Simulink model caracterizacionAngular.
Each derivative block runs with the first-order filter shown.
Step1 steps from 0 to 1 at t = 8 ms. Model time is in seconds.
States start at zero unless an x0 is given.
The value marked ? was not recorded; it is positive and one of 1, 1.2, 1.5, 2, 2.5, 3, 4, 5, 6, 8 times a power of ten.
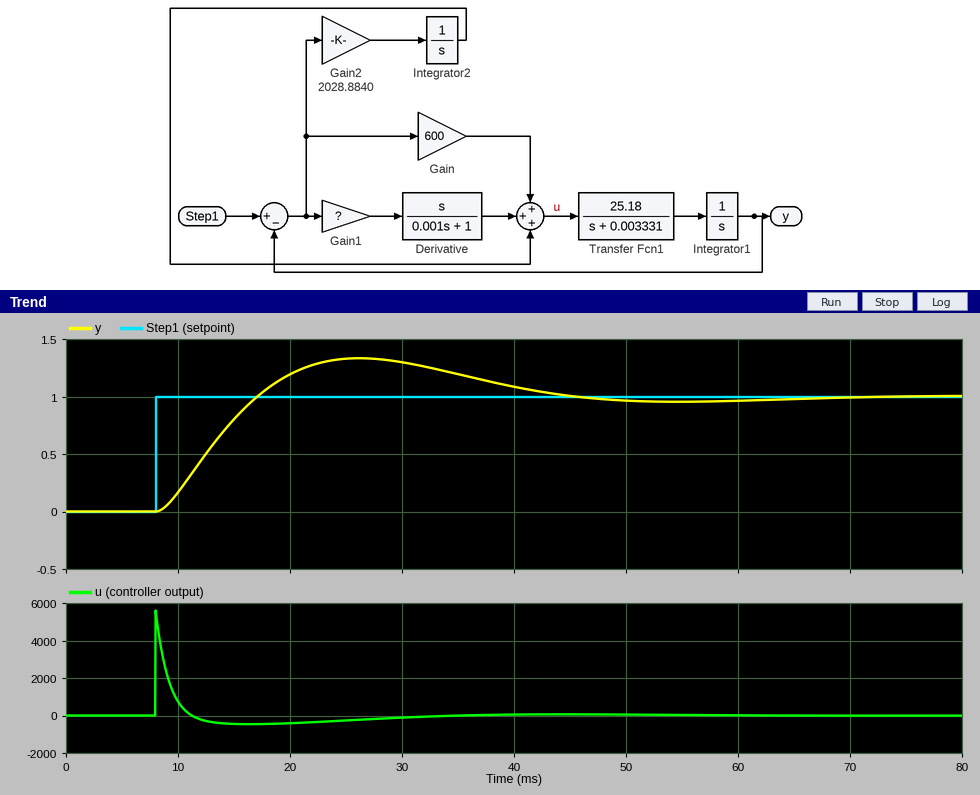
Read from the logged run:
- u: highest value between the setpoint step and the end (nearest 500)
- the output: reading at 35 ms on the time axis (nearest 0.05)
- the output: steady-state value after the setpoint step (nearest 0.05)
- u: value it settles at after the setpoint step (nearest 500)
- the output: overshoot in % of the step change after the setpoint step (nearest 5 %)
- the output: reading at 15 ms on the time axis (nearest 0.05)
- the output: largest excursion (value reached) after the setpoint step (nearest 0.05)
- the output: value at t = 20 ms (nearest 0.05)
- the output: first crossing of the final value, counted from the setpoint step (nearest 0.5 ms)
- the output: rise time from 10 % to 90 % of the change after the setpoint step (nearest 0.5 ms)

5500
1.20
1.00
0
35 %
0.80
1.35
1.20
9.0 ms
6.5 ms
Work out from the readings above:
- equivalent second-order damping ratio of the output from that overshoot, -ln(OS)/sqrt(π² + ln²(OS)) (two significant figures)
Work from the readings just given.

0.32
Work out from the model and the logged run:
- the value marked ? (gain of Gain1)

5
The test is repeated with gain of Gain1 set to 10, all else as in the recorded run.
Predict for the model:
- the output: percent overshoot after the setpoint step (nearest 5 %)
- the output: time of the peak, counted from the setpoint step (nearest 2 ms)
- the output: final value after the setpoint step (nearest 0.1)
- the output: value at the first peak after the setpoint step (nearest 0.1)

15 %
12 ms
1.0
1.2
